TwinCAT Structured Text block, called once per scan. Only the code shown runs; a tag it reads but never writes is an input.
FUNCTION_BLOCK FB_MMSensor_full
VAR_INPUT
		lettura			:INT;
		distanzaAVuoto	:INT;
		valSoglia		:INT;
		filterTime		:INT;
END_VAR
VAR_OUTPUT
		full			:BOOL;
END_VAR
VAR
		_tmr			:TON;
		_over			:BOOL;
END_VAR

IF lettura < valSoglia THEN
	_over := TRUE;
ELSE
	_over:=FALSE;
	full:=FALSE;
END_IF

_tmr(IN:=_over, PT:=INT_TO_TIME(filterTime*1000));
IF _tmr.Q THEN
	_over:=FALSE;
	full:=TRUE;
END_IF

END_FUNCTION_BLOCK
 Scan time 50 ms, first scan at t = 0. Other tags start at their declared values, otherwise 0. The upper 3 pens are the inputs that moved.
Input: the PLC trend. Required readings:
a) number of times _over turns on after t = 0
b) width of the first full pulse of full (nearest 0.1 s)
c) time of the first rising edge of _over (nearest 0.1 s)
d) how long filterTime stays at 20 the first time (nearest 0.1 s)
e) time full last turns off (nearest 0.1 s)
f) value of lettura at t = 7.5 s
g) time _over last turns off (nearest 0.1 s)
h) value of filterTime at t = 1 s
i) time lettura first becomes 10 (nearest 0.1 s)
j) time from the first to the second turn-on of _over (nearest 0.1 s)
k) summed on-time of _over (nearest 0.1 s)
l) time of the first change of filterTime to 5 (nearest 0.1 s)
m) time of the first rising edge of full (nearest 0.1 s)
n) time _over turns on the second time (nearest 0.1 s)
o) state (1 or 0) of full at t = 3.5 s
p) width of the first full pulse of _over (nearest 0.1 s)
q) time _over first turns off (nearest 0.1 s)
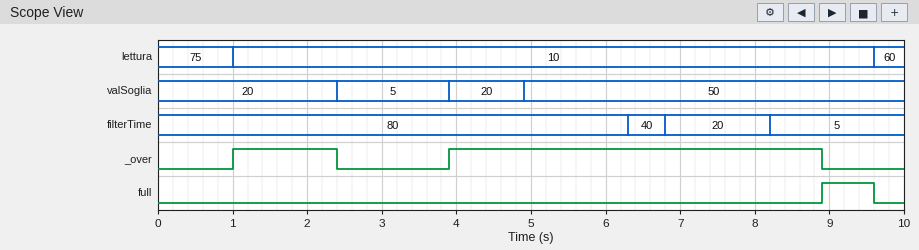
2
0.7 s
1.0 s
1.4 s
9.6 s
10
8.9 s
80
1.0 s
2.9 s
6.4 s
8.2 s
8.9 s
3.9 s
0
1.4 s
2.4 s
